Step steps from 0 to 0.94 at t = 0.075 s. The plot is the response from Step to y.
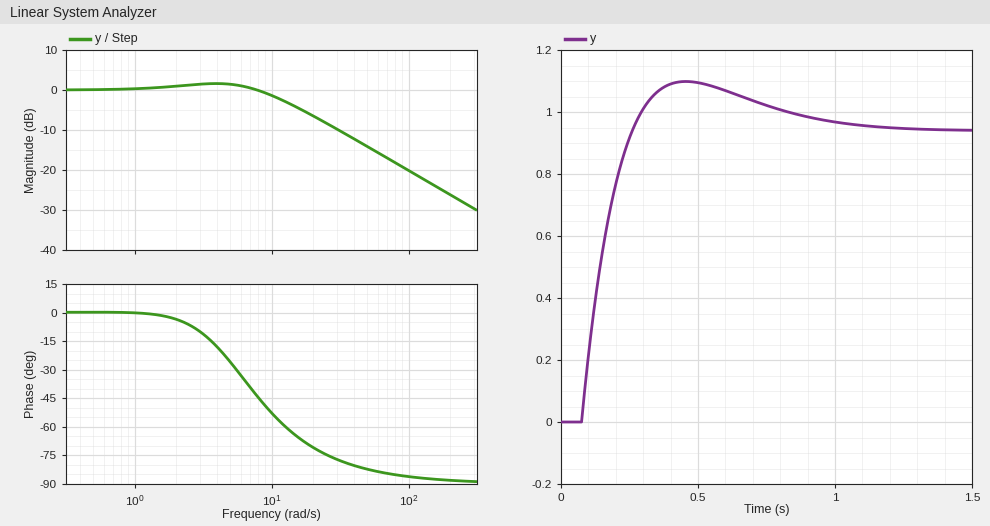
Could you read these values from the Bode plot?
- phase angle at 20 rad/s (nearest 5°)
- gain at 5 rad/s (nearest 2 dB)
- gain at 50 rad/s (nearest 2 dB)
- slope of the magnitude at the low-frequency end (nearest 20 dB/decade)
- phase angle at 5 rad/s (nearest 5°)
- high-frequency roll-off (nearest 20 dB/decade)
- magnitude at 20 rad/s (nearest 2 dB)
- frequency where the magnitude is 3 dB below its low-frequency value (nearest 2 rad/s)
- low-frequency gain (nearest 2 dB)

-70°
2 dB
-14 dB
0 dB/decade
-25°
-20 dB/decade
-6 dB
12 rad/s
0 dB
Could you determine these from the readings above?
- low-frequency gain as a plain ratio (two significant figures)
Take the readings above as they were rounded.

1.0
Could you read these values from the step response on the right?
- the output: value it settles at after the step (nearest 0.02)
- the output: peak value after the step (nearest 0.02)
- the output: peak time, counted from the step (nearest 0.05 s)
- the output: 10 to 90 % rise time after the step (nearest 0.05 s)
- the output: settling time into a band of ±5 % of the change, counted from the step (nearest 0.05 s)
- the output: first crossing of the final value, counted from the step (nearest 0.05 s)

0.94
1.10
0.40 s
0.15 s
0.80 s
0.20 s
